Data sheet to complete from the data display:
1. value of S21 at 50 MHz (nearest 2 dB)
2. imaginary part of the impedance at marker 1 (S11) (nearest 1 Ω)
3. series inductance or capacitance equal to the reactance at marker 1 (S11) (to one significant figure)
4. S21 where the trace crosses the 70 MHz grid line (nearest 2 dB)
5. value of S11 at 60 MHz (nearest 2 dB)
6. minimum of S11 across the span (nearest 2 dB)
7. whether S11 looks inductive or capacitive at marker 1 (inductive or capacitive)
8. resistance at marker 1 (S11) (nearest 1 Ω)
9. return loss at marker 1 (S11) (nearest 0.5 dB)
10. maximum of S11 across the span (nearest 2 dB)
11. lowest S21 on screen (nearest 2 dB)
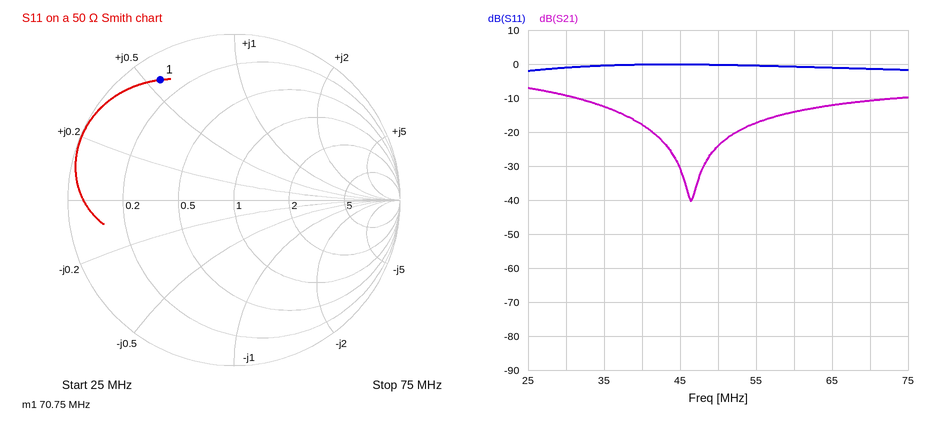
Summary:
-24 dB
+28 Ω
60 nH
-10 dB
0 dB
-2 dB
inductive
5 Ω
1.5 dB
0 dB
-40 dB
